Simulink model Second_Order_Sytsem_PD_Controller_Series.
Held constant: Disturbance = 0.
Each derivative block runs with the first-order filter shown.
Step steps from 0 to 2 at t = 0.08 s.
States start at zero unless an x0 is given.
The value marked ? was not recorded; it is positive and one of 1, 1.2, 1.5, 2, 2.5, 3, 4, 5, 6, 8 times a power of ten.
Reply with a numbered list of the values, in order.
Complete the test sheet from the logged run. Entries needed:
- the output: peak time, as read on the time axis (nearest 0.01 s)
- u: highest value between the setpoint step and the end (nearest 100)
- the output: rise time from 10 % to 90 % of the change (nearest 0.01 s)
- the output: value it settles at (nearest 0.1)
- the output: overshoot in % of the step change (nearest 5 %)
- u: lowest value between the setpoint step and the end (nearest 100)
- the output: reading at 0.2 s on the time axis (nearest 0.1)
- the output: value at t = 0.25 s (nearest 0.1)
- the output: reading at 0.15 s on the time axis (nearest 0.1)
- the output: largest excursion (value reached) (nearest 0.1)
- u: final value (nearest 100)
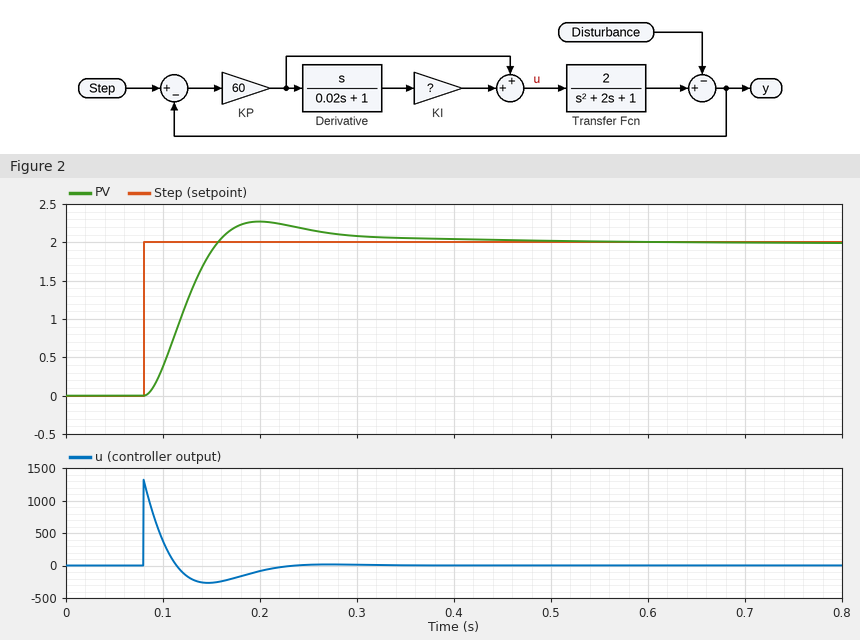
1. 0.20 s
2. 1300
3. 0.05 s
4. 2.0
5. 15 %
6. -300
7. 2.3
8. 2.2
9. 1.9
10. 2.3
11. 0
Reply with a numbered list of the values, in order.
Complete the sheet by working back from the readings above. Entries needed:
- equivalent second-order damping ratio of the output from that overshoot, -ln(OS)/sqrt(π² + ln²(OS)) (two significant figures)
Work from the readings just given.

1. 0.52
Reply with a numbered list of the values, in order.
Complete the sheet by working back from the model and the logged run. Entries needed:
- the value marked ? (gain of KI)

1. 0.2
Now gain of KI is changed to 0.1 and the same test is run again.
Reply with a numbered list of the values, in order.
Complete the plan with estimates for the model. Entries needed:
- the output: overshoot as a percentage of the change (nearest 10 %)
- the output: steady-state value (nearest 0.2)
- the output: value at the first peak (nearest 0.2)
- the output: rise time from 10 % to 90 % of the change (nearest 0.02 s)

1. 20 %
2. 2.0
3. 2.4
4. 0.08 s
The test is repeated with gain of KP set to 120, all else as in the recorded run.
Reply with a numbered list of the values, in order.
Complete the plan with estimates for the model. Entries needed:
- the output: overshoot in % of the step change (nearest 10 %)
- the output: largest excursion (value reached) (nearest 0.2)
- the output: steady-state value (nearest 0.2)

1. 20 %
2. 2.4
3. 2.0
